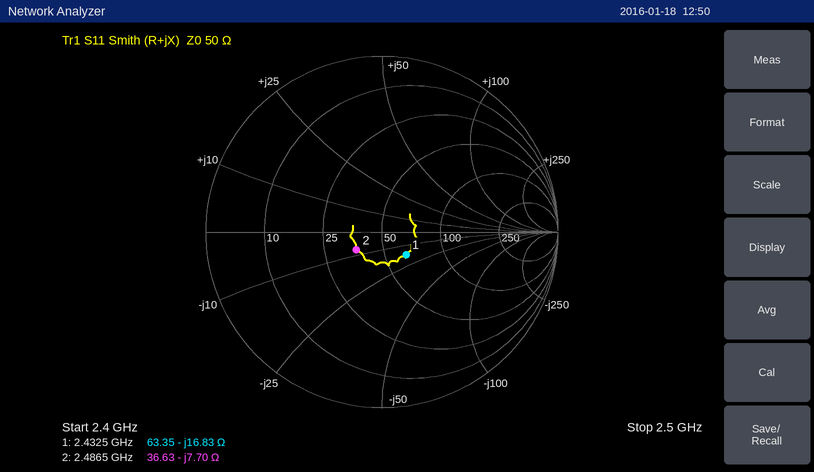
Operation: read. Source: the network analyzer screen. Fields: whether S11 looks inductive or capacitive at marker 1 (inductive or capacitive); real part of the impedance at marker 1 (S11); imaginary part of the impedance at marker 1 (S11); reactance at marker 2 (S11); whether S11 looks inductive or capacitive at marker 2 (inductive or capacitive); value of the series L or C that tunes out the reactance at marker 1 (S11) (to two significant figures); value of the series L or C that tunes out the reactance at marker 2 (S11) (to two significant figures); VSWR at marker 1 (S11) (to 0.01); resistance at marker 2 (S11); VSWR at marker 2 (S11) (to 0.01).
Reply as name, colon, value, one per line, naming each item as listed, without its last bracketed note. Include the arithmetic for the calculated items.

whether S11 looks inductive or capacitive at marker 1: capacitive
real part of the impedance at marker 1: 63.35 Ω
imaginary part of the impedance at marker 1: -16.83 Ω
reactance at marker 2: -7.70 Ω
whether S11 looks inductive or capacitive at marker 2: capacitive
value of the series L or C that tunes out the reactance at marker 1 (S11): L = 16.83 Ω/(2π × 2.4325 GHz) ≈ 1.1 nH
value of the series L or C that tunes out the reactance at marker 2 (S11): L = 7.7 Ω/(2π × 2.4865 GHz) ≈ 493 pH, so 490 pH to two significant figures
VSWR at marker 1 (S11): 1.46
resistance at marker 2: 36.63 Ω
VSWR at marker 2 (S11): 1.43
